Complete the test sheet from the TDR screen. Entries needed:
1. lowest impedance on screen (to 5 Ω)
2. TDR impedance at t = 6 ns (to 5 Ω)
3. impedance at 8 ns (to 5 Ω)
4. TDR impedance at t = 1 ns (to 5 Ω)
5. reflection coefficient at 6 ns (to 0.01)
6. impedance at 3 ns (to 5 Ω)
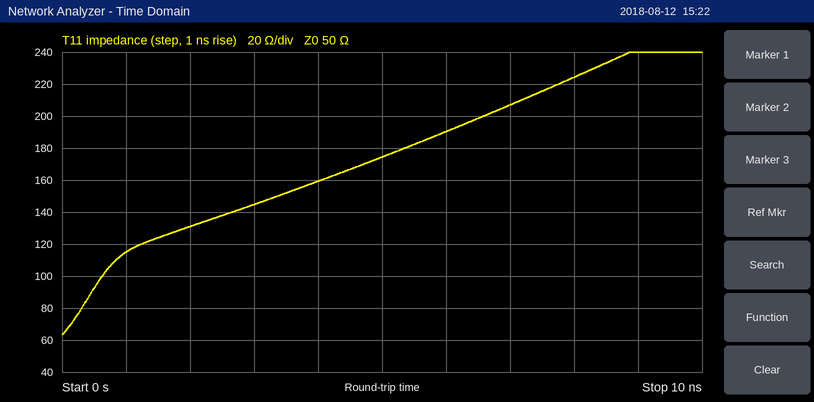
65 Ω
190 Ω
225 Ω
115 Ω
+0.58
145 Ω
